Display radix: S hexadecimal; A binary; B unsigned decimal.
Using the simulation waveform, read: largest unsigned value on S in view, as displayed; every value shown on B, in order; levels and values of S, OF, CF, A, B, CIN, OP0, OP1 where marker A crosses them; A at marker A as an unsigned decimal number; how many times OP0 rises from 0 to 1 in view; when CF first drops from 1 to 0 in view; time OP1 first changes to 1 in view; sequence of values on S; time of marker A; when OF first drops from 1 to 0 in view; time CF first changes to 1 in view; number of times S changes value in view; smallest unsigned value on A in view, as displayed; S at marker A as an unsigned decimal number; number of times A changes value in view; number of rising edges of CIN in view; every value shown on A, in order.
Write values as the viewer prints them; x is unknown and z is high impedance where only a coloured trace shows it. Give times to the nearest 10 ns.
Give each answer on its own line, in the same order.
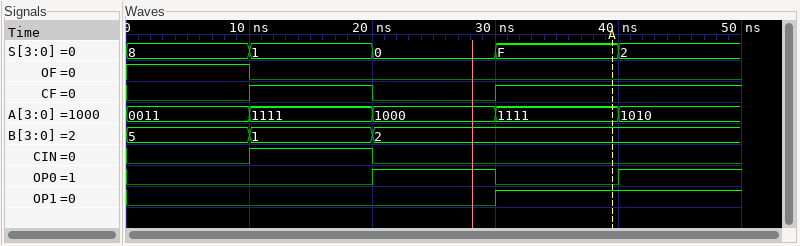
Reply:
F
5, 1, 2
S=F, OF=0, CF=1, A=1111, B=2, CIN=0, OP0=0, OP1=1
15
2
20 ns
30 ns
8, 1, 0, F, 2
40 ns
10 ns
10 ns
4
0011
15
4
1
0011, 1111, 1000, 1111, 1010
